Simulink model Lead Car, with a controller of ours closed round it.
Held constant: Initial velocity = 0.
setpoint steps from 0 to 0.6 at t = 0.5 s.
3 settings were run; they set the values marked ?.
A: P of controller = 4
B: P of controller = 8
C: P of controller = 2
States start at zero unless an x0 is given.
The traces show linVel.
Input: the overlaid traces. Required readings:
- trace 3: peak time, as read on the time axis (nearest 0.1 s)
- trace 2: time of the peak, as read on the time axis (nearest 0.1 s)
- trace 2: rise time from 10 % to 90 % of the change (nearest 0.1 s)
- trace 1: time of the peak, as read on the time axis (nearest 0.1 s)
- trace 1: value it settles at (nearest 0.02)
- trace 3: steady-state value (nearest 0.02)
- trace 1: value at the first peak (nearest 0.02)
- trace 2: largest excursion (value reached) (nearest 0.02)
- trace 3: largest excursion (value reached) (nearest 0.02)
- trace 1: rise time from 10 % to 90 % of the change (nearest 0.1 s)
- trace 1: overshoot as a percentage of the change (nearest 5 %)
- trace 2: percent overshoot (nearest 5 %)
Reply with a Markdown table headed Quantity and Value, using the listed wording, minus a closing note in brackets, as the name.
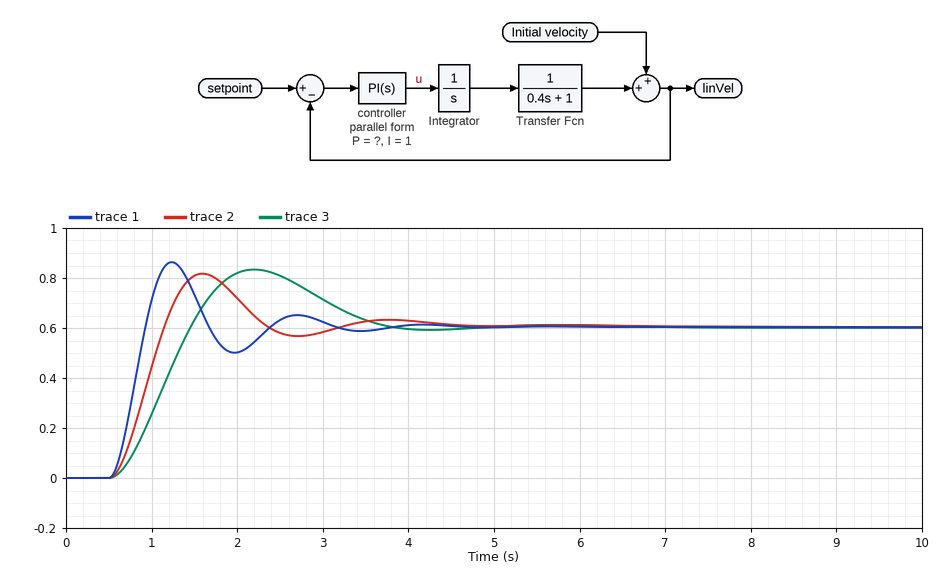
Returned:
| Quantity | Value |
|---|---|
| trace 3: peak time, as read on the time axis | 2.2 s |
| trace 2: time of the peak, as read on the time axis | 1.6 s |
| trace 2: rise time from 10 % to 90 % of the change | 0.4 s |
| trace 1: time of the peak, as read on the time axis | 1.2 s |
| trace 1: value it settles at | 0.60 |
| trace 3: steady-state value | 0.60 |
| trace 1: value at the first peak | 0.86 |
| trace 2: largest excursion (value reached) | 0.82 |
| trace 3: largest excursion (value reached) | 0.84 |
| trace 1: rise time from 10 % to 90 % of the change | 0.3 s |
| trace 1: overshoot as a percentage of the change | 45 % |
| trace 2: percent overshoot | 35 % |
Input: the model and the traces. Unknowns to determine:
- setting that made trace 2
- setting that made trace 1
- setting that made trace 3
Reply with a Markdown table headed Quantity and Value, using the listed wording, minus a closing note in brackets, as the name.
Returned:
| Quantity | Value |
|---|---|
| setting that made trace 2 | A |
| setting that made trace 1 | B |
| setting that made trace 3 | C |
